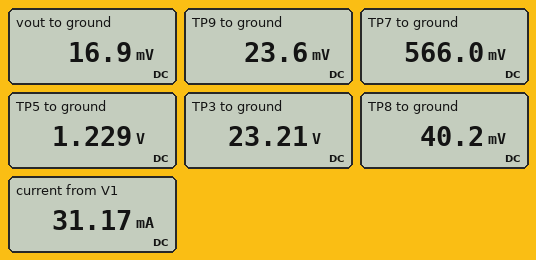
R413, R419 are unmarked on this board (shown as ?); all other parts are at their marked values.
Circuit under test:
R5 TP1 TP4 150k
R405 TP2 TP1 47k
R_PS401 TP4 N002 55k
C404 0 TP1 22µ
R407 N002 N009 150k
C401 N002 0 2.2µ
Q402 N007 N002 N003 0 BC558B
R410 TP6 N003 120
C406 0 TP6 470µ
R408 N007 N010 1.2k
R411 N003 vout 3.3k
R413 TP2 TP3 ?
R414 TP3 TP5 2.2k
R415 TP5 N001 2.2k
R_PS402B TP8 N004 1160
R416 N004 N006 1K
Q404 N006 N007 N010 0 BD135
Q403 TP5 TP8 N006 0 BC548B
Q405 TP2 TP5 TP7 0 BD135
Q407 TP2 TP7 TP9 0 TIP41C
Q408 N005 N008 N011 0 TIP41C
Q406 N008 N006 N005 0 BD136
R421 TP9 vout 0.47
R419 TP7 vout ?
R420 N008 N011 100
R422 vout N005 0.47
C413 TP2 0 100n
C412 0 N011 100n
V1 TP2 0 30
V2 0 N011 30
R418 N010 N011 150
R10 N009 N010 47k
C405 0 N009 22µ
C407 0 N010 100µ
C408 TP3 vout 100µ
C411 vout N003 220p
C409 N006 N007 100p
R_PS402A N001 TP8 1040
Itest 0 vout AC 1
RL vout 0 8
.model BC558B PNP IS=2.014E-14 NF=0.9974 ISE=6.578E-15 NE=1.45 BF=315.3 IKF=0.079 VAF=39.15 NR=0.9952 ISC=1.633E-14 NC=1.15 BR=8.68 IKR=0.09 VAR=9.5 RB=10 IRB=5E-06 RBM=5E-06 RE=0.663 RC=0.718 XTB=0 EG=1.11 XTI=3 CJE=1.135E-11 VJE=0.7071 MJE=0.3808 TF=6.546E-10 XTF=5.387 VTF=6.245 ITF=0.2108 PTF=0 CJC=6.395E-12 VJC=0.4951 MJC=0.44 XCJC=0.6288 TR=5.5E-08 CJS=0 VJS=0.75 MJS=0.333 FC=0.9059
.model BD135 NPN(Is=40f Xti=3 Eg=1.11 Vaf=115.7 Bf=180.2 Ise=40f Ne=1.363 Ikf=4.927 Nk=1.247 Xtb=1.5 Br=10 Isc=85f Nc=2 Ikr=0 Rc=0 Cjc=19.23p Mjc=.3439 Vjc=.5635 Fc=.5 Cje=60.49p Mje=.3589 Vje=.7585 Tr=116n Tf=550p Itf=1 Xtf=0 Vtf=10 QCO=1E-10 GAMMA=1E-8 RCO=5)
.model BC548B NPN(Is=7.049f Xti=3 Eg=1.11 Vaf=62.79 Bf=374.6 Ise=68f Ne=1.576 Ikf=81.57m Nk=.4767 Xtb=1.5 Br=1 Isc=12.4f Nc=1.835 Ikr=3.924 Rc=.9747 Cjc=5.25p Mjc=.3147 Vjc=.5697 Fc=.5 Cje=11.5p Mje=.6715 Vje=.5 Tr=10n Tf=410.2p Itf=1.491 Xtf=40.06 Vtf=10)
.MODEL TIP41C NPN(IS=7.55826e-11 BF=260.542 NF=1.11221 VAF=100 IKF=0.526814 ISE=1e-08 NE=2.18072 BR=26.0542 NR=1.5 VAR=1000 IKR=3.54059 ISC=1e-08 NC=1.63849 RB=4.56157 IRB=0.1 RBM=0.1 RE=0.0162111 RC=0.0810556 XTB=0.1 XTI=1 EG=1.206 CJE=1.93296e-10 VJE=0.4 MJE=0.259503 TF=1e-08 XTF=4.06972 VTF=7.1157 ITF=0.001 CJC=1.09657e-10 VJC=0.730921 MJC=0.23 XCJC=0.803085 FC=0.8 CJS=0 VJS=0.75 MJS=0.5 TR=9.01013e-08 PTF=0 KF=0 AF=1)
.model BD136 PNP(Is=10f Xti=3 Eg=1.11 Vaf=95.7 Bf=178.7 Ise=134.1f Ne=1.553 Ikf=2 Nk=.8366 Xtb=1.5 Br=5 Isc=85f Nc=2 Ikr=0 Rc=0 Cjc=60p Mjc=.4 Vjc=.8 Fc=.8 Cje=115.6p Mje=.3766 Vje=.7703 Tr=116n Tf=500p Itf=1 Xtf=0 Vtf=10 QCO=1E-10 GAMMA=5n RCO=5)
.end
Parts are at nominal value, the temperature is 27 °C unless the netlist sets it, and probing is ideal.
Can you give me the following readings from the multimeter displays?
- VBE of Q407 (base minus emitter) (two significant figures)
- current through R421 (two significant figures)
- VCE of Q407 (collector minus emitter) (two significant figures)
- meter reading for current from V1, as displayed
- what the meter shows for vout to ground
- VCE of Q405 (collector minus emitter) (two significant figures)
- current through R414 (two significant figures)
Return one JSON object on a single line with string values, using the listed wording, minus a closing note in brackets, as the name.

{"VBE of Q407 (base minus emitter)": "540 mV", "current through R421": "14 mA", "VCE of Q407 (collector minus emitter)": "30 V", "meter reading for current from V1, as displayed": "31.17 mA", "what the meter shows for vout to ground": "16.9 mV", "VCE of Q405 (collector minus emitter)": "29 V", "current through R414": "10 mA"}
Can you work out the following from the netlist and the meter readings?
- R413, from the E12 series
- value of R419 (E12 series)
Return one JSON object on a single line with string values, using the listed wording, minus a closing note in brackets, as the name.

{"R413, from the E12 series": "680 Ω", "value of R419": "82 Ω"}
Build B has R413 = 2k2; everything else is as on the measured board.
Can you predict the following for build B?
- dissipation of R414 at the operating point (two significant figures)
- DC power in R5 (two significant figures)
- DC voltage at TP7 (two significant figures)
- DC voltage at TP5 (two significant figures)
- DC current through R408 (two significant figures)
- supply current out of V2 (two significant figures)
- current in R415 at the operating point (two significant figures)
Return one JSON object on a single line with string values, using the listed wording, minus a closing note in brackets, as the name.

{"dissipation of R414 at the operating point": "97 mW", "DC power in R5": "2.6 mW", "DC voltage at TP7": "110 mV", "DC voltage at TP5": "770 mV", "DC current through R408": "550 µA", "supply current out of V2": "59 mA", "current in R415 at the operating point": "350 µA"}
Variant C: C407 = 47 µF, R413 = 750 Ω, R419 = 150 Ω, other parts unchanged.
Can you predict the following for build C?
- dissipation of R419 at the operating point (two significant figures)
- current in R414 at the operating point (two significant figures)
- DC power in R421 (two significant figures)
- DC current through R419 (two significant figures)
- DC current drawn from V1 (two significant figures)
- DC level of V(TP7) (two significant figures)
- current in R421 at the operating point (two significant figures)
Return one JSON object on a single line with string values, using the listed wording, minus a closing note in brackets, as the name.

{"dissipation of R419 at the operating point": "2.1 mW", "current in R414 at the operating point": "9.8 mA", "DC power in R421": "150 µW", "DC current through R419": "3.7 mA", "DC current drawn from V1": "32 mA", "DC level of V(TP7)": "550 mV", "current in R421 at the operating point": "18 mA"}
